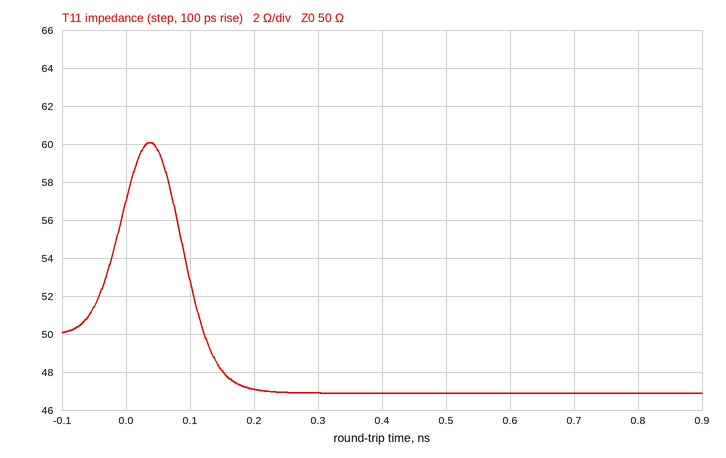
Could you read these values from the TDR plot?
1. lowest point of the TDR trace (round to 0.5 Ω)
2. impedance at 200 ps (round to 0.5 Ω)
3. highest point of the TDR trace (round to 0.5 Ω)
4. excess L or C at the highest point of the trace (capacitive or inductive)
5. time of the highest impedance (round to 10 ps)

47.0 Ω
47.0 Ω
60.0 Ω
inductive
40 ps
